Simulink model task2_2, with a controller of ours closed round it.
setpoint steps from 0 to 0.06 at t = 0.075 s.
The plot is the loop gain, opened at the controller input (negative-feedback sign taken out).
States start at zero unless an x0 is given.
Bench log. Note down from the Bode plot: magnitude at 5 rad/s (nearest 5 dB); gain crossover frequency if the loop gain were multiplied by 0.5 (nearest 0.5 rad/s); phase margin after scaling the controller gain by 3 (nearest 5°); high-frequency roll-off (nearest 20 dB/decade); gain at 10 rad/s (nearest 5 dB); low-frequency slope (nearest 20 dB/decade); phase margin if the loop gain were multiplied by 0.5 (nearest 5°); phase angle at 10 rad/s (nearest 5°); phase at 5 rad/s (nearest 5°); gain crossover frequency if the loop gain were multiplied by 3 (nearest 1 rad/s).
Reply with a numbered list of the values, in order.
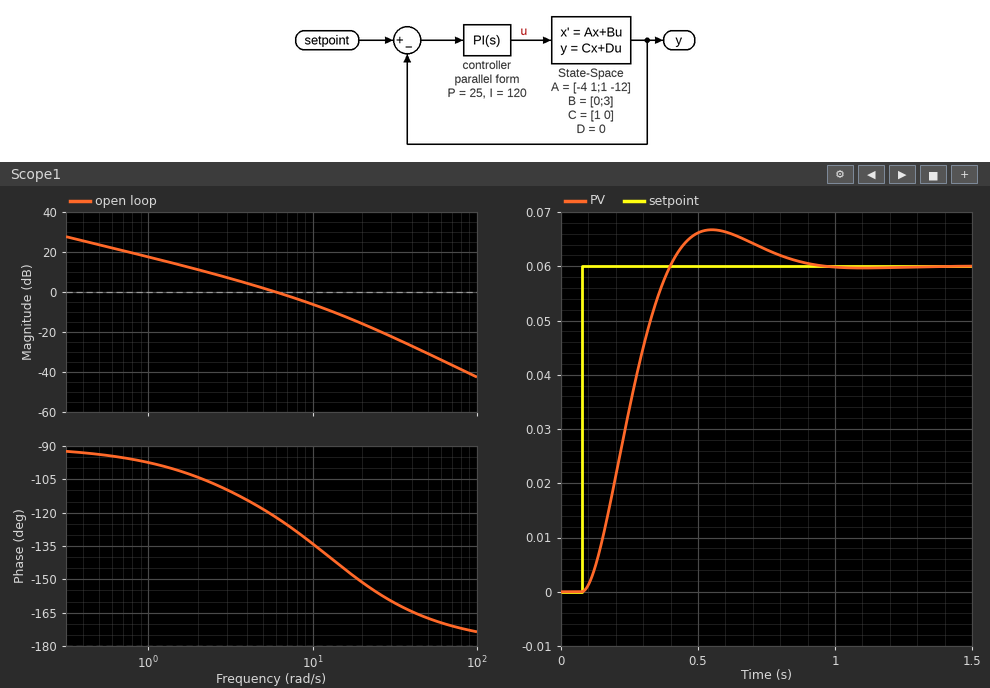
1. 0 dB
2. 3.5 rad/s
3. 40°
4. -40 dB/decade
5. -5 dB
6. -20 dB/decade
7. 70°
8. -135°
9. -120°
10. 13 rad/s
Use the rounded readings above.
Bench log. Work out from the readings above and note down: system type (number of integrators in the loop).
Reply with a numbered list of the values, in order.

1. 1
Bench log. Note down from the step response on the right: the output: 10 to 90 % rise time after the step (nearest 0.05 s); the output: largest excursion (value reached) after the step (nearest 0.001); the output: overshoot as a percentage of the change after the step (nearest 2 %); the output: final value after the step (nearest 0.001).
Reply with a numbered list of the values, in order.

1. 0.20 s
2. 0.067
3. 12 %
4. 0.060
